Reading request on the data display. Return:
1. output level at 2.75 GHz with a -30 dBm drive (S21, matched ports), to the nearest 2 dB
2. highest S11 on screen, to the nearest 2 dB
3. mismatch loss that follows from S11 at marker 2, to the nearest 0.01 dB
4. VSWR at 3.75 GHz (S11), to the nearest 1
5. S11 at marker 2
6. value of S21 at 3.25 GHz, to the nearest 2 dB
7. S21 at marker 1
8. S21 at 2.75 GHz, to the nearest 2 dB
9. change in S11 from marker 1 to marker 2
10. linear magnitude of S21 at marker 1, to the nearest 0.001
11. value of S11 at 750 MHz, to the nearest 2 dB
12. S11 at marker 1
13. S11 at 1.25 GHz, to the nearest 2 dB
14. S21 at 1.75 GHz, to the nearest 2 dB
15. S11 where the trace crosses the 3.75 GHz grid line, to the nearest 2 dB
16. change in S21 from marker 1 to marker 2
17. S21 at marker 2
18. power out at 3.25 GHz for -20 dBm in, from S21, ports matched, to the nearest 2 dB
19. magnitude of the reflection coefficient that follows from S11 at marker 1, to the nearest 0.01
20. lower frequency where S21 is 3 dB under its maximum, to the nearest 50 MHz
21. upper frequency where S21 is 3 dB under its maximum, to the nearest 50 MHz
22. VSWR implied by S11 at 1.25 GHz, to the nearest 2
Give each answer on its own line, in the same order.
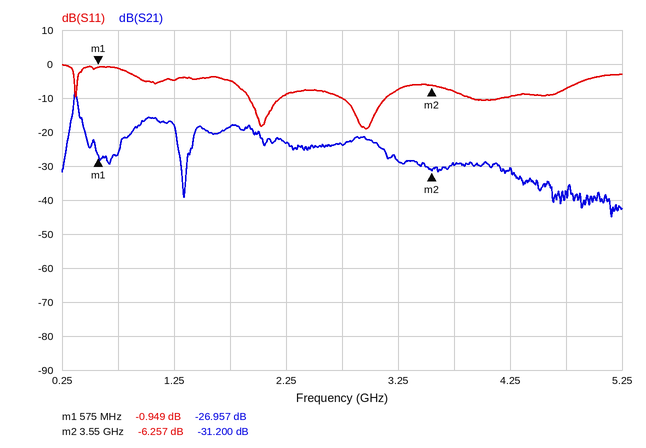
-54 dBm
0 dB
1.17 dB
2
-6.257 dB
-28 dB
-26.957 dB
-24 dB
-5.308 dB
0.045
-2 dB
-0.949 dB
-4 dB
-18 dB
-8 dB
-4.243 dB
-31.200 dB
-48 dBm
0.90
350 MHz
400 MHz
4
